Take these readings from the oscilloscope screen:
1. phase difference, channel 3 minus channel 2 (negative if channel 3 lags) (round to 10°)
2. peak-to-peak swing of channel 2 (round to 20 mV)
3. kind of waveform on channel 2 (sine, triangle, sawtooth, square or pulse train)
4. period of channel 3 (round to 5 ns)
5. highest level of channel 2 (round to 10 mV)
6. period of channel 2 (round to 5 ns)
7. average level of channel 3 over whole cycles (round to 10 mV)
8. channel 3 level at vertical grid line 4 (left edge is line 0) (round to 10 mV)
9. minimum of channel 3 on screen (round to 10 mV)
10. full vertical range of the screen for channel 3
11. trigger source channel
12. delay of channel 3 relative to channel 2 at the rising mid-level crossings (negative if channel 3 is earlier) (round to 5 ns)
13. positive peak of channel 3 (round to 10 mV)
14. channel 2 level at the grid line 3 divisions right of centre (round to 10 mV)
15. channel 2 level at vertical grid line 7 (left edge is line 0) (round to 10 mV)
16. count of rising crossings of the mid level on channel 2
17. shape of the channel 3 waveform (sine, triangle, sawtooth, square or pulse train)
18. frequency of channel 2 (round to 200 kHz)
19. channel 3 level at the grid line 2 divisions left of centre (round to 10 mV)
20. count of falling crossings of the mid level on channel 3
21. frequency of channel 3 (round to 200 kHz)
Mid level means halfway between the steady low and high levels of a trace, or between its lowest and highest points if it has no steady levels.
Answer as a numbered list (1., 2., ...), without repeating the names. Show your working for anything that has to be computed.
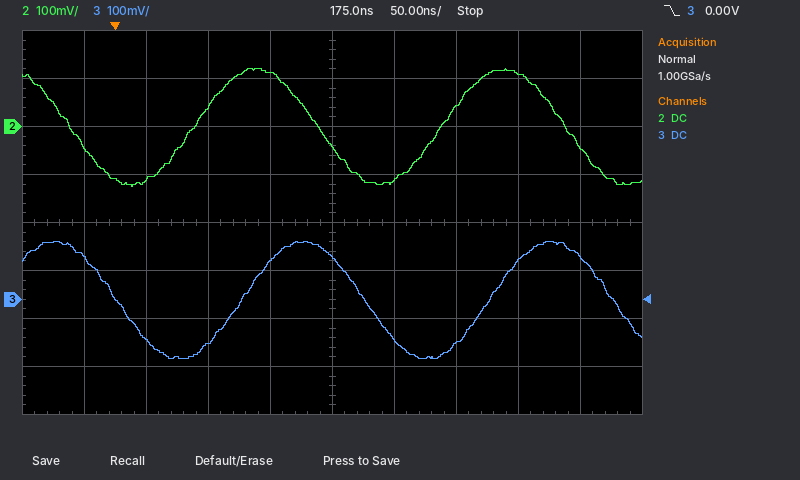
1. −360° × (+40 ns) / 200 ns ≈ -72.0°, so -70° to the nearest 10°
2. 240 mV
3. sine
4. 200 ns
5. 120 mV
6. 200 ns
7. (120 mV + (-120 mV)) / 2 ≈ 0 mV
8. 80 mV
9. -120 mV
10. 800 mV
11. channel 3
12. +40 ns
13. 120 mV
14. 110 mV
15. 40 mV
16. 2
17. sine
18. 1 / 200 ns ≈ 5.0 MHz
19. -90 mV
20. 3
21. 1 / 200 ns ≈ 5.0 MHz
